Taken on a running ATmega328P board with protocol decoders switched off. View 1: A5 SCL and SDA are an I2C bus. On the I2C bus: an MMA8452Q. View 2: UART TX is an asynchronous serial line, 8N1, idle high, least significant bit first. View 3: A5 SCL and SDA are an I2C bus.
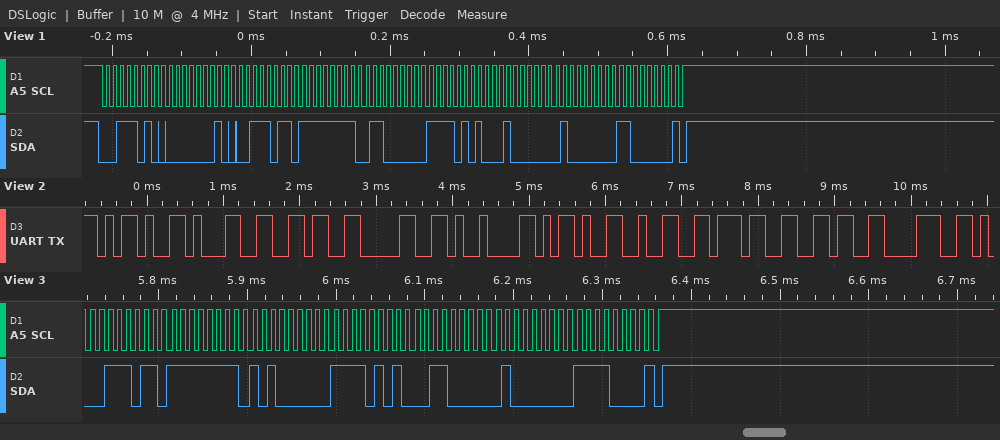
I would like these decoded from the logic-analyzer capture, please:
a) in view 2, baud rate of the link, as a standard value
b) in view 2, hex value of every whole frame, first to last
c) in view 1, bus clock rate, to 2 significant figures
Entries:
9600 baud
2D 31 36 30 09 2D 32 37 36 38
100 kHz
